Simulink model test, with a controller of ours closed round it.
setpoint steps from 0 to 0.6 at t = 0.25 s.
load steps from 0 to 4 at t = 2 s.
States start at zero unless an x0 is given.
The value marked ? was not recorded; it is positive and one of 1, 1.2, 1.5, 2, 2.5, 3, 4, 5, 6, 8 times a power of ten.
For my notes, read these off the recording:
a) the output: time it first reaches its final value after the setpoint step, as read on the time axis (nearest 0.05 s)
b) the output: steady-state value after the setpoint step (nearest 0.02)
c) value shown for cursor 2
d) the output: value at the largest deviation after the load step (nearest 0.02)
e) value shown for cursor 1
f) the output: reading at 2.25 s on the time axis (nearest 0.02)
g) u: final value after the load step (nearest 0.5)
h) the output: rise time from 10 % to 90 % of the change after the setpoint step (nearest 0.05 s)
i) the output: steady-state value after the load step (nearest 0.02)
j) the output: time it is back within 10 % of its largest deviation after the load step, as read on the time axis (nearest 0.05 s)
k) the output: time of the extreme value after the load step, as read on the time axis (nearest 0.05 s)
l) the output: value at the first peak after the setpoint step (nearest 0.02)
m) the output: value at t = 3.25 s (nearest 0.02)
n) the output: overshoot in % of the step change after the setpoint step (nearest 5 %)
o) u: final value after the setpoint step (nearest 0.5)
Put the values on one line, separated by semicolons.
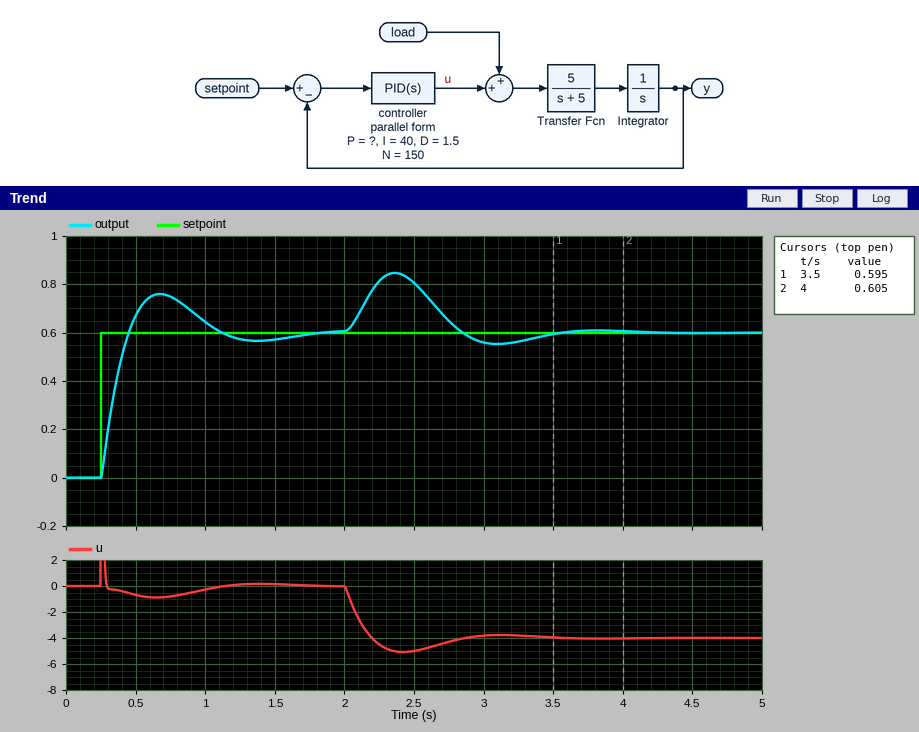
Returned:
0.45 s; 0.60; 0.605; 0.84; 0.595; 0.82; -4.0; 0.15 s; 0.60; 3.35 s; 2.35 s; 0.76; 0.56; 25 %; 0.0
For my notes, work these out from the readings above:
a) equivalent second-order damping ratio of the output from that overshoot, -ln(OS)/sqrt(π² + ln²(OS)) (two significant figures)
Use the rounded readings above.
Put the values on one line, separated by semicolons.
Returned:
0.40
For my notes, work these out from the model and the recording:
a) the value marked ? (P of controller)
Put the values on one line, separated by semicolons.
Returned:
12
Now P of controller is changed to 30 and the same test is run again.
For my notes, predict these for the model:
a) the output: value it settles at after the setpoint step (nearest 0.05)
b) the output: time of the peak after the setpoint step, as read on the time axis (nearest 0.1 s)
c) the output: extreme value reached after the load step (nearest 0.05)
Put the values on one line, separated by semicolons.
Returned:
0.60; 0.5 s; 0.75
